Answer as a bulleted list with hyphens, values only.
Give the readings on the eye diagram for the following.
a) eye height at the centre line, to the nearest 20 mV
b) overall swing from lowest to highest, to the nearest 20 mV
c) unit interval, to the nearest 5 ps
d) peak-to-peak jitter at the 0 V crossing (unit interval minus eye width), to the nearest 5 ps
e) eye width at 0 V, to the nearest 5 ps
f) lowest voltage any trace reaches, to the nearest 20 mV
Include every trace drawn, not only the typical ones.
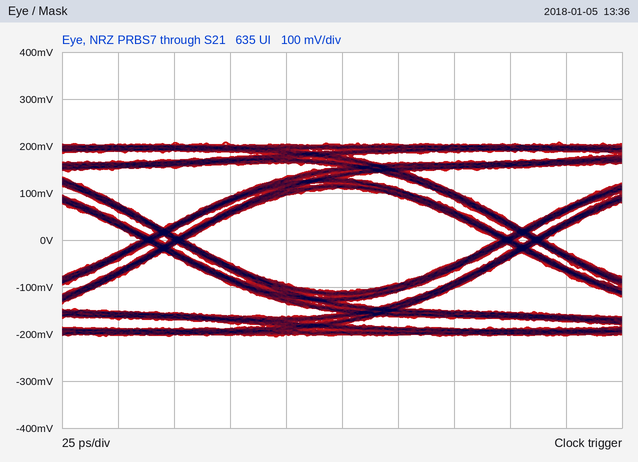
- 220 mV
- 420 mV
- 160 ps
- 20 ps
- 140 ps
- -200 mV
